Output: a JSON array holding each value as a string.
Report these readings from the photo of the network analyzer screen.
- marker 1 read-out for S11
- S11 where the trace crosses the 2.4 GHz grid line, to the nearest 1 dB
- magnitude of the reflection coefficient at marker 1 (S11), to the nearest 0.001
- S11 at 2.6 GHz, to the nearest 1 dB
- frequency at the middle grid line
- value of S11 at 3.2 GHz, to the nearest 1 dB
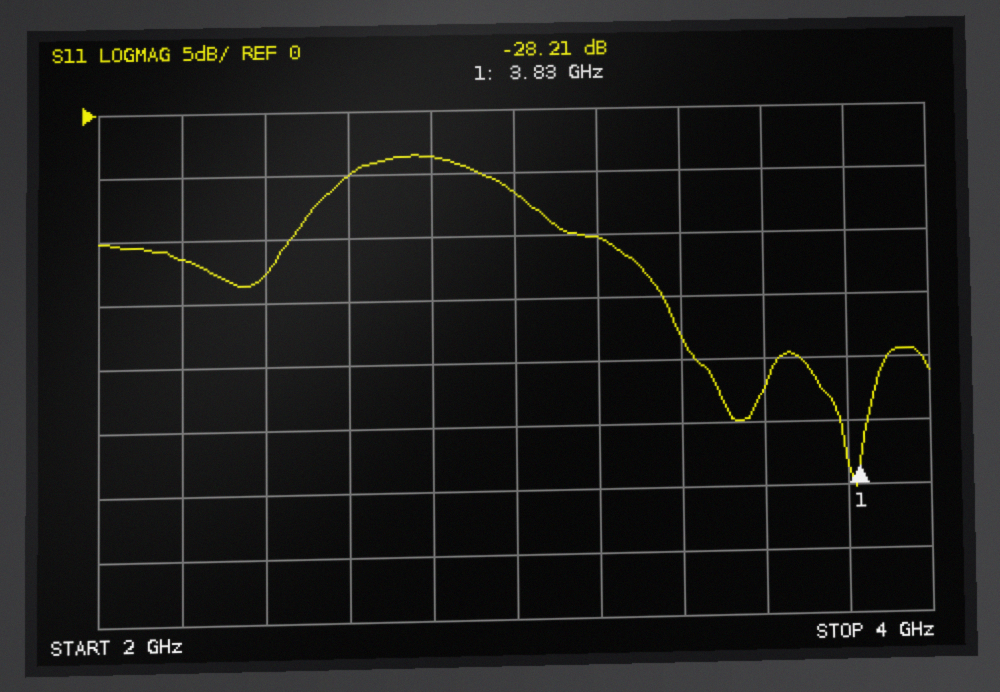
["-28.21 dB", "-13 dB", "0.039", "-5 dB", "3 GHz", "-10 dB"]
